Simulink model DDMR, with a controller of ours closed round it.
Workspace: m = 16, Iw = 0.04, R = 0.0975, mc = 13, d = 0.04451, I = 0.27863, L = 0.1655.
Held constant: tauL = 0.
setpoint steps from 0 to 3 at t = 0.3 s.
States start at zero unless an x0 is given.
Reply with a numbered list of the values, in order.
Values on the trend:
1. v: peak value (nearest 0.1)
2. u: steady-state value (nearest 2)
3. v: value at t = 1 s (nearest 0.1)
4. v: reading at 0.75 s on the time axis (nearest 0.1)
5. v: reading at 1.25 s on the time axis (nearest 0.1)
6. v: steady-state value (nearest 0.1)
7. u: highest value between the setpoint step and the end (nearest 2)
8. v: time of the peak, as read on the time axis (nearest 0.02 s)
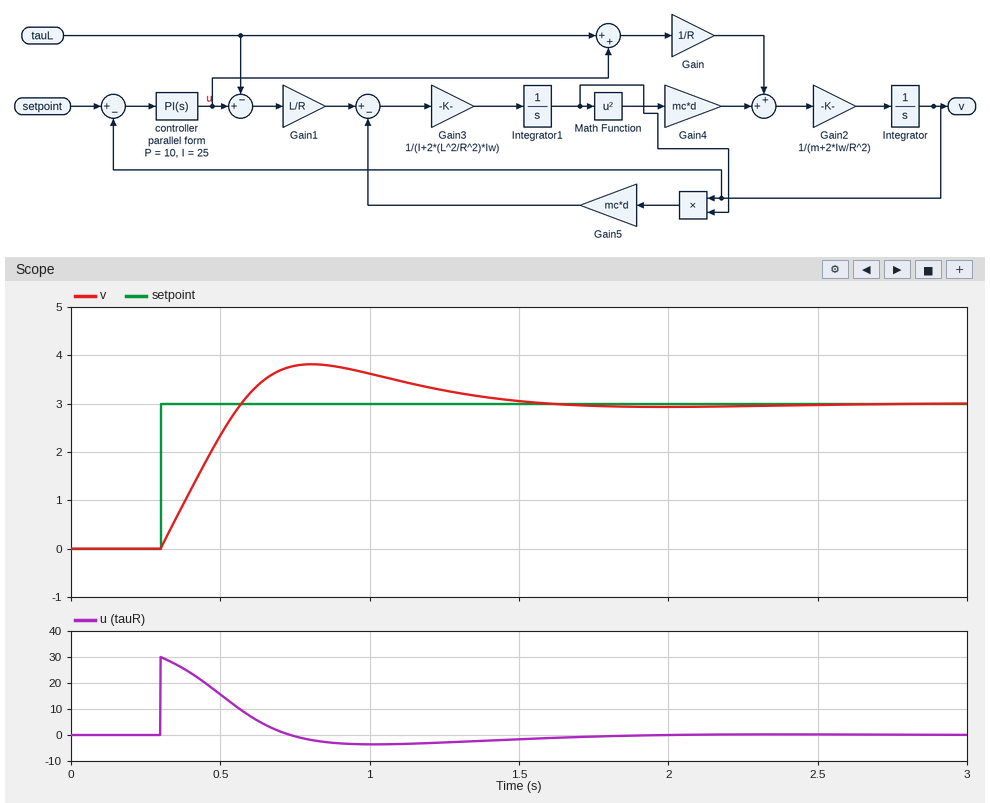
1. 3.8
2. 0
3. 3.6
4. 3.8
5. 3.3
6. 3.0
7. 30
8. 0.80 s
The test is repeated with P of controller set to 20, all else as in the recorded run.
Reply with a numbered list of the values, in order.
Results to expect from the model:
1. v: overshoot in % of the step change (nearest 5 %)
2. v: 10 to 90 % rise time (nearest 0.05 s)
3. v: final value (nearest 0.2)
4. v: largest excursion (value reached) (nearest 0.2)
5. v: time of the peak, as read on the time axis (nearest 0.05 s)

1. 15 %
2. 0.15 s
3. 3.0
4. 3.4
5. 0.65 s
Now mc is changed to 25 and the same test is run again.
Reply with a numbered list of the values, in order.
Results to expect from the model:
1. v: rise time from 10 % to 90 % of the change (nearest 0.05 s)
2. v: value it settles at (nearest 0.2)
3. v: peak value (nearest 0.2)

1. 0.20 s
2. 3.0
3. 3.6
